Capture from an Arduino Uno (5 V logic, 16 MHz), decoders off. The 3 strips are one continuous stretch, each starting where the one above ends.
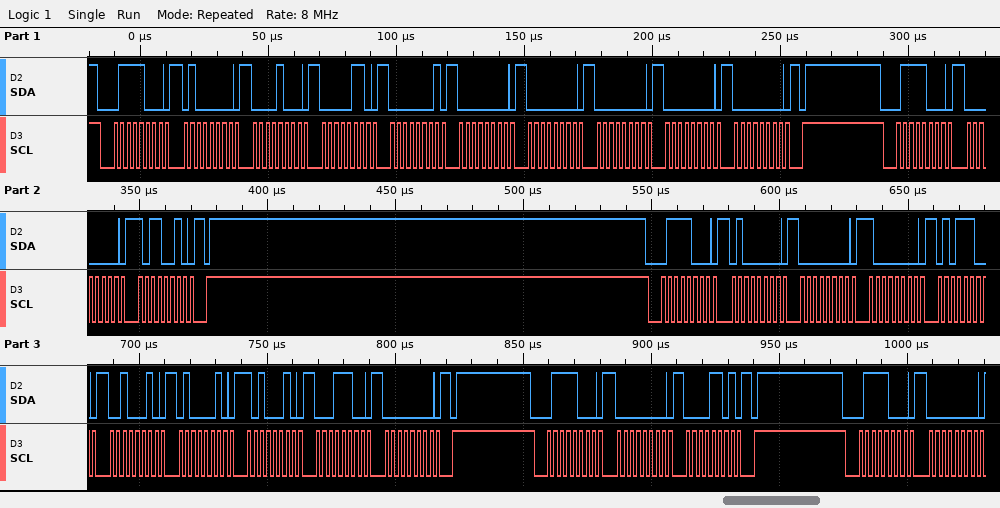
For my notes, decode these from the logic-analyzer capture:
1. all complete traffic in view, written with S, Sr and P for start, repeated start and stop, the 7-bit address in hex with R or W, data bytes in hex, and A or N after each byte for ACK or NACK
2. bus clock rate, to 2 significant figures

S 3CW A 40 A 08 A 06 A 01 A 00 A 00 A 00 A 00 A 00 A P S 3CW A 00 A B2 A P S 3CW A 40 A 00 A 80 A 5C A 22 A 42 A A2 A 1C A 00 A P S 3CW A 00 A 0D A P S 3CW A 00 A
400 kHz
